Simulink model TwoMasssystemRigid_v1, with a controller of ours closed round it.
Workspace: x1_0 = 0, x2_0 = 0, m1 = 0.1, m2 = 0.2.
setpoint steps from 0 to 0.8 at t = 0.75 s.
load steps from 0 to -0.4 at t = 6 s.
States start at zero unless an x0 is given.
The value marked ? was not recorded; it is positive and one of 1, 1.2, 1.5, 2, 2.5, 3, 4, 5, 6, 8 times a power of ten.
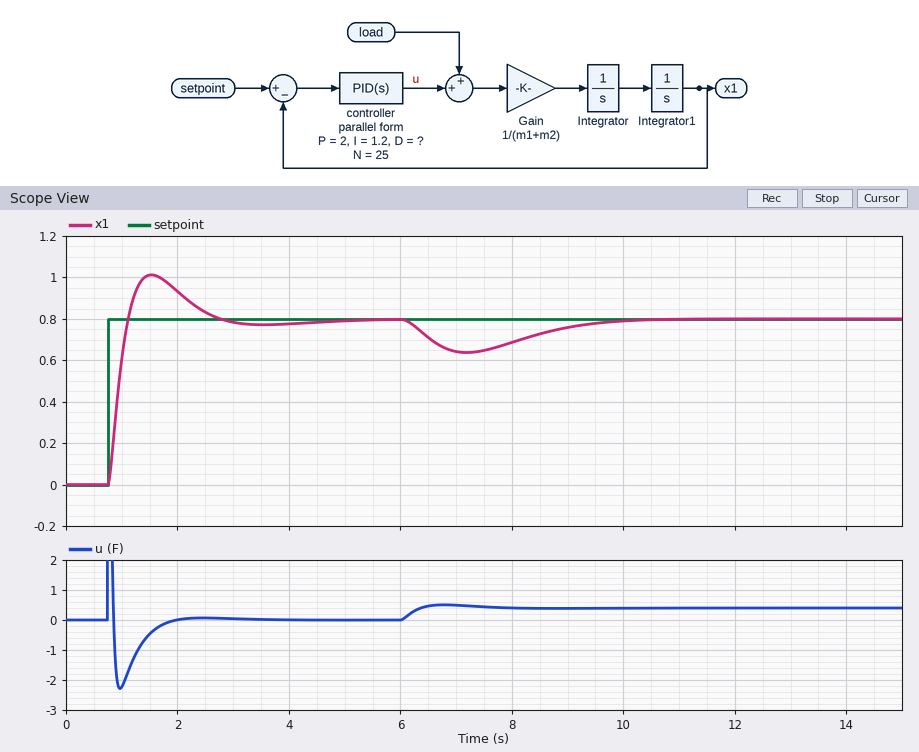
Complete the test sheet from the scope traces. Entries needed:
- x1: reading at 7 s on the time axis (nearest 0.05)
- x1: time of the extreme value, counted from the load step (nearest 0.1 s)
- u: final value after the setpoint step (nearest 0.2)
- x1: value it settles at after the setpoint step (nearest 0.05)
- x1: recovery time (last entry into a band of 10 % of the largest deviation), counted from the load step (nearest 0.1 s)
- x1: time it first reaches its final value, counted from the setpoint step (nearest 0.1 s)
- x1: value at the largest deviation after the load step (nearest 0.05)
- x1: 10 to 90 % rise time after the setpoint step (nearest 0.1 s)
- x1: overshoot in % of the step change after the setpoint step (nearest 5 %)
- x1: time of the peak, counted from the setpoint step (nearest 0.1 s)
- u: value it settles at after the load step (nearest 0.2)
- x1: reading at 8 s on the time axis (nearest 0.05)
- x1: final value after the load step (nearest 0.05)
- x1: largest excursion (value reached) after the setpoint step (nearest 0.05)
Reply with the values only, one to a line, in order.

0.65
1.2 s
0.0
0.80
3.7 s
0.4 s
0.65
0.3 s
25 %
0.8 s
0.4
0.70
0.80
1.00
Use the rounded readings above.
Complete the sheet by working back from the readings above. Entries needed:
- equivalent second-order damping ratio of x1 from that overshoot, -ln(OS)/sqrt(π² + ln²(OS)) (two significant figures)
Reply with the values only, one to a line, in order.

0.40
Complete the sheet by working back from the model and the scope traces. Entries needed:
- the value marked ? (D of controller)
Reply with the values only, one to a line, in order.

1.2
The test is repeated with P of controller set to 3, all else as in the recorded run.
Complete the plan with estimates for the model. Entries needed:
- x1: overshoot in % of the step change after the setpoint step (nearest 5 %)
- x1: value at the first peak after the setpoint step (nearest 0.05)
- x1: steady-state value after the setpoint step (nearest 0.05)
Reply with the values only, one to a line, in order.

30 %
1.05
0.80
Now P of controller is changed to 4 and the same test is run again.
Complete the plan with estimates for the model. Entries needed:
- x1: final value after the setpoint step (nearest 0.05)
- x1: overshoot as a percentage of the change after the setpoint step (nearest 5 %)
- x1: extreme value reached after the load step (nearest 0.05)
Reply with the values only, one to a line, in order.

0.80
35 %
0.70
